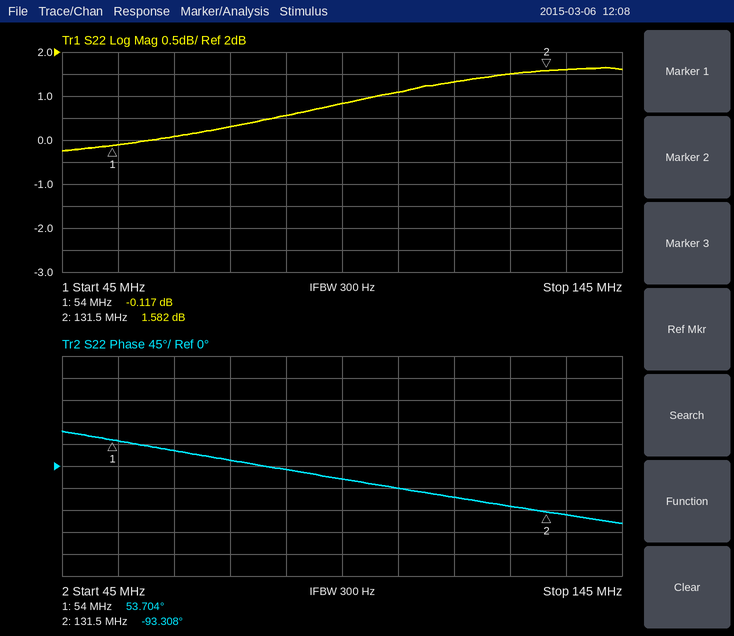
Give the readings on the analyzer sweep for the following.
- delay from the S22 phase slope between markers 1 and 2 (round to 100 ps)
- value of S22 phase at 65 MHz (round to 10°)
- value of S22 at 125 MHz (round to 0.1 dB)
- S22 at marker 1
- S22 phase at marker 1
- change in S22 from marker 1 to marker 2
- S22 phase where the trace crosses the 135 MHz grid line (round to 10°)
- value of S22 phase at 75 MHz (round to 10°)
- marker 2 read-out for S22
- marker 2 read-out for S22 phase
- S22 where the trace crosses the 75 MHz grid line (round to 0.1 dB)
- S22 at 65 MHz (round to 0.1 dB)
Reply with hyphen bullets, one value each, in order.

- 5.3 ns
- 30°
- 1.5 dB
- -0.117 dB
- 53.704°
- 1.699 dB
- -100°
- 10°
- 1.582 dB
- -93.308°
- 0.3 dB
- 0.1 dB
